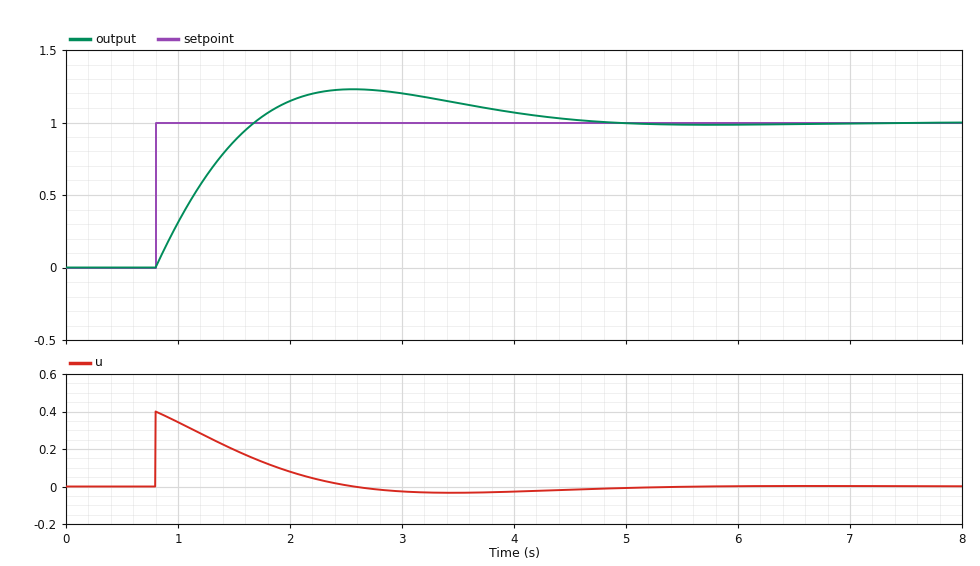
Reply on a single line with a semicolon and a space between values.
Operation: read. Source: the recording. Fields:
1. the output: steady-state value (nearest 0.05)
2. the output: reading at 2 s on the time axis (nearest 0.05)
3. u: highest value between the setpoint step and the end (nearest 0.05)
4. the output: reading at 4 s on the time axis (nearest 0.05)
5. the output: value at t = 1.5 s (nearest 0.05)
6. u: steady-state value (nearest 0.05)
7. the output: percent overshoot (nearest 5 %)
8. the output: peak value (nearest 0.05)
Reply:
1.00; 1.15; 0.40; 1.05; 0.85; 0.00; 25 %; 1.25
